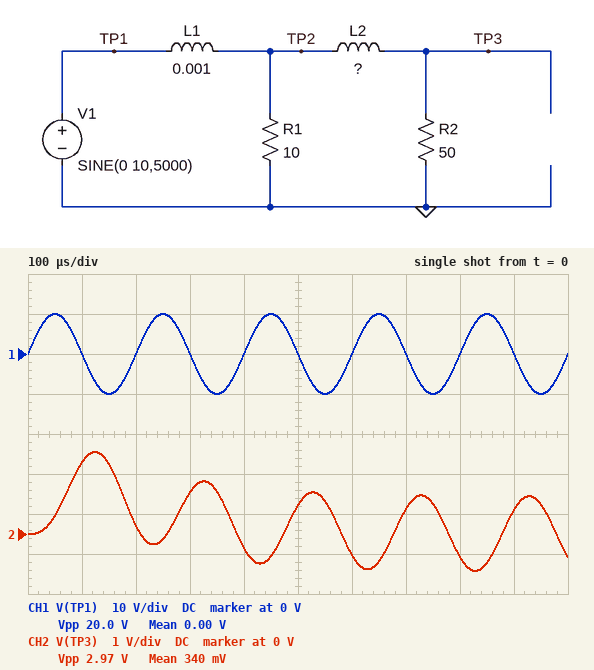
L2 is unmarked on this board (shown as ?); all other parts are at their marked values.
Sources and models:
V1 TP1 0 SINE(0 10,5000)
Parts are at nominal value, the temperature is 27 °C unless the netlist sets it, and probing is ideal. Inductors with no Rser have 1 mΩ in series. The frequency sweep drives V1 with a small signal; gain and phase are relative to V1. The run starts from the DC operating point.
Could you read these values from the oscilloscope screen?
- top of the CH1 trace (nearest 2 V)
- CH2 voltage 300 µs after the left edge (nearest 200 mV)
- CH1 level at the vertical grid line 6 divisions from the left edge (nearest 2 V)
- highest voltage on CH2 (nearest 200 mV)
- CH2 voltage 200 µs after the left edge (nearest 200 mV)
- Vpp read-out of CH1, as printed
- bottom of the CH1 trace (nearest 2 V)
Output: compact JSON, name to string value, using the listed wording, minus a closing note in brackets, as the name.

{"top of the CH1 trace": "10 V", "CH2 voltage 300 µs after the left edge": "1.0 V", "CH1 level at the vertical grid line 6 divisions from the left edge": "0 V", "highest voltage on CH2": "2.0 V", "CH2 voltage 200 µs after the left edge": "200 mV", "Vpp read-out of CH1, as printed": "20.0 V", "bottom of the CH1 trace": "-10 V"}
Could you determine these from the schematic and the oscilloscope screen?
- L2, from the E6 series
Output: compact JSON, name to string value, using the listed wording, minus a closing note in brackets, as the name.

{"L2, from the E6 series": "4.7 mH"}
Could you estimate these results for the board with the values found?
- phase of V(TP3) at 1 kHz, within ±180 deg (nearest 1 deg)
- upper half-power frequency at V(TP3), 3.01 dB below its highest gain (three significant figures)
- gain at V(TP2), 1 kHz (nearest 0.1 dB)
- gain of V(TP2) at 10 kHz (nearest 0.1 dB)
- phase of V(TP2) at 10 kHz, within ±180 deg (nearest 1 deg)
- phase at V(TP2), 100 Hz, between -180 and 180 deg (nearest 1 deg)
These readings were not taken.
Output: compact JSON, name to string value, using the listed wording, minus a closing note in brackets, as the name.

{"phase of V(TP3) at 1 kHz, within ±180 deg": "-65 deg", "upper half-power frequency at V(TP3), 3.01 dB below its highest gain": "920 Hz", "gain at V(TP2), 1 kHz": "-2.1 dB", "gain of V(TP2) at 10 kHz": "-16.2 dB", "phase of V(TP2) at 10 kHz, within ±180 deg": "-79 deg", "phase at V(TP2), 100 Hz, between -180 and 180 deg": "-4 deg"}
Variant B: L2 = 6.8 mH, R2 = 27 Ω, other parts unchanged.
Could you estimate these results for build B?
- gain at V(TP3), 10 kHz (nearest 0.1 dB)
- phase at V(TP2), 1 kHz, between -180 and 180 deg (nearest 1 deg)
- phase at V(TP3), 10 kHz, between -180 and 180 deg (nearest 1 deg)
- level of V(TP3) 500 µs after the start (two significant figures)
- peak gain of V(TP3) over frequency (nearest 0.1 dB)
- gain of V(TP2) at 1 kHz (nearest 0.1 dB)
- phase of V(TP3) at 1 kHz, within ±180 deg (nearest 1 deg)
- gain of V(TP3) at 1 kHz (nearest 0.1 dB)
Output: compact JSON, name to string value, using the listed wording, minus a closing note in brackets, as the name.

{"gain at V(TP3), 10 kHz": "-40.1 dB", "phase at V(TP2), 1 kHz, between -180 and 180 deg": "-32 deg", "phase at V(TP3), 10 kHz, between -180 and 180 deg": "-166 deg", "level of V(TP3) 500 µs after the start": "440 mV", "peak gain of V(TP3) over frequency": "0 dB", "gain of V(TP2) at 1 kHz": "-2.3 dB", "phase of V(TP3) at 1 kHz, within ±180 deg": "-90 deg", "gain of V(TP3) at 1 kHz": "-7.8 dB"}
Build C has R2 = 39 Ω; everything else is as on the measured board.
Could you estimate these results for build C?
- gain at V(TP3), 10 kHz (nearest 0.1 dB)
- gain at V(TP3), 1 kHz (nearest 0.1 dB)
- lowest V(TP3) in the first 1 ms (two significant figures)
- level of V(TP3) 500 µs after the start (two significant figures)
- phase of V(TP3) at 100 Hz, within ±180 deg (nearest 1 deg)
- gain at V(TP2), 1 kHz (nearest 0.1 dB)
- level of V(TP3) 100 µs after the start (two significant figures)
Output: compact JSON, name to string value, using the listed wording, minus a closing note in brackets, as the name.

{"gain at V(TP3), 10 kHz": "-33.8 dB", "gain at V(TP3), 1 kHz": "-4.3 dB", "lowest V(TP3) in the first 1 ms": "-720 mV", "level of V(TP3) 500 µs after the start": "600 mV", "phase of V(TP3) at 100 Hz, within ±180 deg": "-9 deg", "gain at V(TP2), 1 kHz": "-2.3 dB", "level of V(TP3) 100 µs after the start": "1.5 V"}
